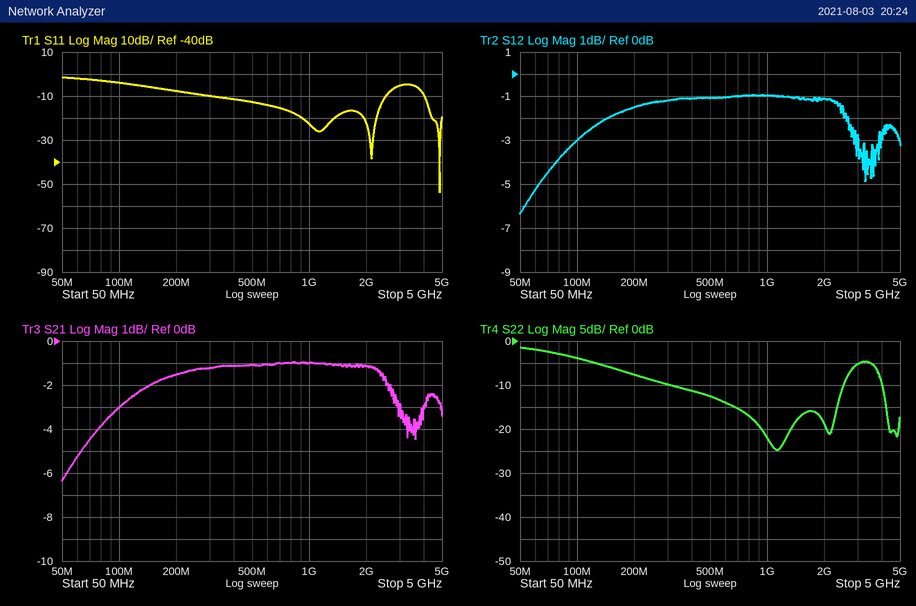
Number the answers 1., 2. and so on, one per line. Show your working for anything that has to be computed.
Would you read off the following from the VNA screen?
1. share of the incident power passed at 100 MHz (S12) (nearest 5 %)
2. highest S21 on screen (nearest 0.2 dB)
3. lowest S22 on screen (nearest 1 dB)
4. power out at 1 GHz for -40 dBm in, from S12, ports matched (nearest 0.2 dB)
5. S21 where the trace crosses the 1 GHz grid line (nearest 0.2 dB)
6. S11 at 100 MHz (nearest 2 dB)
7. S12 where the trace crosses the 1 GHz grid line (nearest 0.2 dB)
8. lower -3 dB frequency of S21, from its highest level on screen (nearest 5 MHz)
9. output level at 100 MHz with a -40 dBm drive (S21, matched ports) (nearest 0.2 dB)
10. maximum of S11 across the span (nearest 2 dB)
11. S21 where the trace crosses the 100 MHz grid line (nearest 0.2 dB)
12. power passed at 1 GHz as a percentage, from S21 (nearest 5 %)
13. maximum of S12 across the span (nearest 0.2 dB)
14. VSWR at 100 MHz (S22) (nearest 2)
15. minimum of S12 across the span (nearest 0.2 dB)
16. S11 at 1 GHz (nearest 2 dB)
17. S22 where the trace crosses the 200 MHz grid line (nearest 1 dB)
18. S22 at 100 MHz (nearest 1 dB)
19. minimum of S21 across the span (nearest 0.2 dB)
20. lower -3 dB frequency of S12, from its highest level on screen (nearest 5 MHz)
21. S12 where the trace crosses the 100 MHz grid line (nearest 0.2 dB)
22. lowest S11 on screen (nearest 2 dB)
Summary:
1. 10^(-3/10) ≈ 50 %
2. -1.0 dB
3. -25 dB
4. -40 dBm + (-1.0 dB) = -41.0 dBm
5. -1.0 dB
6. -4 dB
7. -1.0 dB
8. 80 MHz
9. -40 dBm + (-3.0 dB) = -43.0 dBm
10. -2 dB
11. -3.0 dB
12. 10^(-1/10) ≈ 79.4 %, so 80 % to the nearest 5 %
13. -1.0 dB
14. |Γ| = 10^(-4/20) = 0.6310; VSWR = (1 + 0.6310)/(1 − 0.6310) ≈ 4
15. -6.4 dB
16. -22 dB
17. -8 dB
18. -4 dB
19. -6.4 dB
20. 80 MHz
21. -3.0 dB
22. -54 dB
